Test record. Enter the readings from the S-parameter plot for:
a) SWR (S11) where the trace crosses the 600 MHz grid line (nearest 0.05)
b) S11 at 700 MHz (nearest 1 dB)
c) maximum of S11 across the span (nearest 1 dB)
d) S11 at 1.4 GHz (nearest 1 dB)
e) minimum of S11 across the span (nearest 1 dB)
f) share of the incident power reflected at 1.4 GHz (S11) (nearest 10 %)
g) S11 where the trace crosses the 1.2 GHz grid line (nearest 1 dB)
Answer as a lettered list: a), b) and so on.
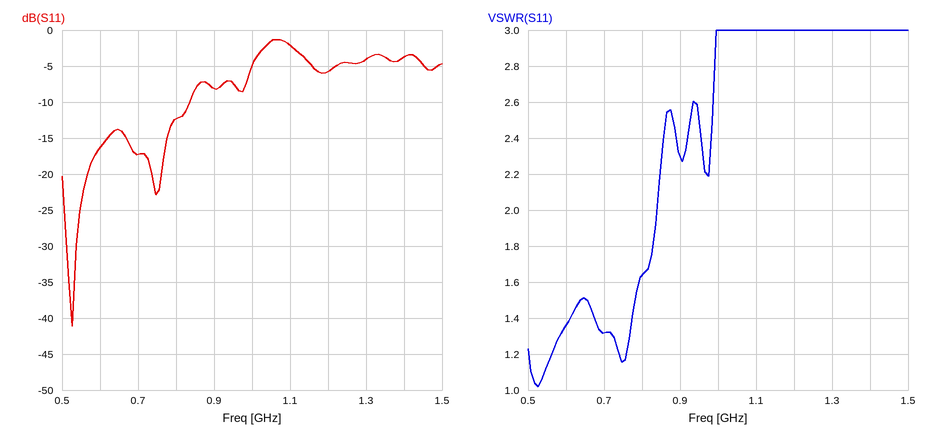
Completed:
a) 1.35
b) -17 dB
c) -1 dB
d) -4 dB
e) -41 dB
f) 40 %
g) -6 dB
